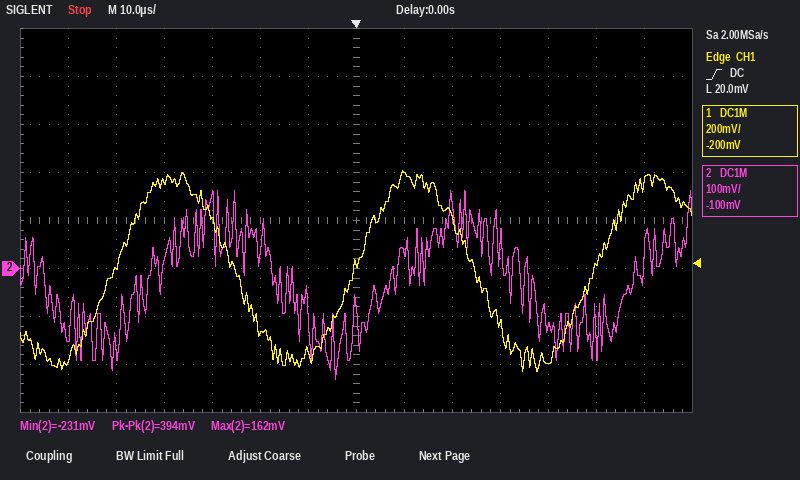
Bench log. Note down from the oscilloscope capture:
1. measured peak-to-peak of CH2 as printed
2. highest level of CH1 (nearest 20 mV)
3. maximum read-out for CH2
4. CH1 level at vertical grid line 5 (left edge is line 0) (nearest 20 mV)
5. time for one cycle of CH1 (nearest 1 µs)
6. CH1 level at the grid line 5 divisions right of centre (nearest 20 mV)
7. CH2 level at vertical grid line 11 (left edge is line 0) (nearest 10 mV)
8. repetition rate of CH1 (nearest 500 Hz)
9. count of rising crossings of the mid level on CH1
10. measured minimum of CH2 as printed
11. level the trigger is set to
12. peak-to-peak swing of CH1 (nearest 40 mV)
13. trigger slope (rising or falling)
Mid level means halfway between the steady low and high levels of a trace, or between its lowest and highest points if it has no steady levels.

394 mV
400 mV
162 mV
-280 mV
50 µs
20 mV
-120 mV
20.0 kHz
3
-231 mV
20.0 mV
840 mV
rising
